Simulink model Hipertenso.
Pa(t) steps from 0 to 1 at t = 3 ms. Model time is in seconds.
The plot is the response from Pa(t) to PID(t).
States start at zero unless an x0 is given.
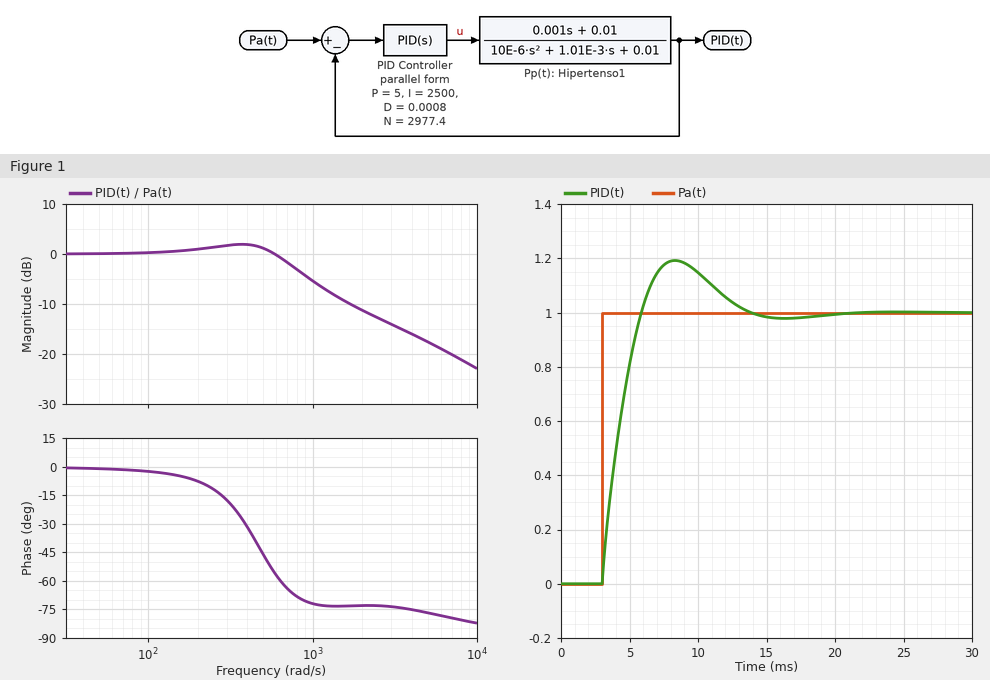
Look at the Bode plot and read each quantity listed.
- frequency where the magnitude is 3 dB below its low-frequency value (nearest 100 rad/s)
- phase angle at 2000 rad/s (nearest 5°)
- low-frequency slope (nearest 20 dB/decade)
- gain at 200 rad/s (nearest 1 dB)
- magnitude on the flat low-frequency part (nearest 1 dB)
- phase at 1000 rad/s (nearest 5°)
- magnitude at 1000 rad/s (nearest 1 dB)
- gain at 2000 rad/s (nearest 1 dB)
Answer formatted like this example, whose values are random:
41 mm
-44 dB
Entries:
800 rad/s
-75°
0 dB/decade
1 dB
0 dB
-70°
-5 dB
-11 dB
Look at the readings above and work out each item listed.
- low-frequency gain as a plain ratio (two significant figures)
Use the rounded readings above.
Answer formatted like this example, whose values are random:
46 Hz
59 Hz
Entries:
1.0
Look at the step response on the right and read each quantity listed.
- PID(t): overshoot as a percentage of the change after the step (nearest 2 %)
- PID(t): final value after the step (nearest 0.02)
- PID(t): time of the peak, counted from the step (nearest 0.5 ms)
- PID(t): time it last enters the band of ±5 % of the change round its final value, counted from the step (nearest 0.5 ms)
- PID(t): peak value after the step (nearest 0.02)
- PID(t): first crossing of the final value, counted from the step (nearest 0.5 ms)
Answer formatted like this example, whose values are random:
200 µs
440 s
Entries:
20 %
1.00
5.5 ms
9.0 ms
1.20
3.0 ms
